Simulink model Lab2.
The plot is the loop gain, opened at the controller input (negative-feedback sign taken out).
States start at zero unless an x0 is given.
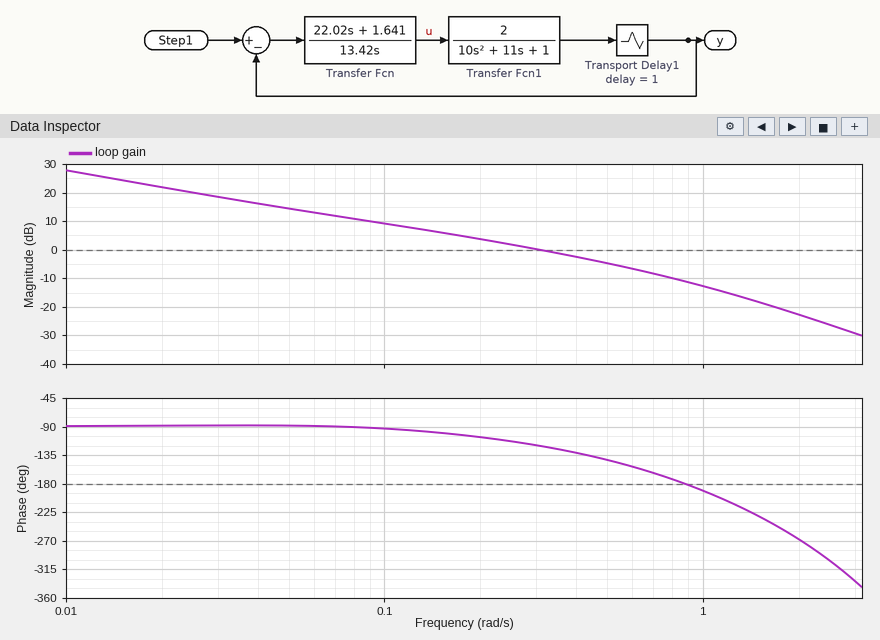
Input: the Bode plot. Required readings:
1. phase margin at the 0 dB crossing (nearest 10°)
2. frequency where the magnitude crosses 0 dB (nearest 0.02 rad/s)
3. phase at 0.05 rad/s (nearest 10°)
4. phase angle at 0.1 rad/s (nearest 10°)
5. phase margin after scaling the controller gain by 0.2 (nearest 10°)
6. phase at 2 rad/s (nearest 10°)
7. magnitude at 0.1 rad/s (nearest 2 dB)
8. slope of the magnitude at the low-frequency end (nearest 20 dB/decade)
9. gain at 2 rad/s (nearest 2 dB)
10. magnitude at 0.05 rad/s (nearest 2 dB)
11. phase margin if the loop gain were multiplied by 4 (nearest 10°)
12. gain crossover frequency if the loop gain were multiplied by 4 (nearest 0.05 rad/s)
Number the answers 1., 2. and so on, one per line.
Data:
1. 60°
2. 0.30 rad/s
3. -90°
4. -90°
5. 90°
6. -270°
7. 10 dB
8. -20 dB/decade
9. -22 dB
10. 14 dB
11. -10°
12. 0.95 rad/s
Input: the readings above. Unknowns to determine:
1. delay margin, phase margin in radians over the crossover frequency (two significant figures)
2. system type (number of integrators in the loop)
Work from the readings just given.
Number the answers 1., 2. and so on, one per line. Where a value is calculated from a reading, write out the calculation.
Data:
1. 60 × π / 180 / 0.3 = 3.5 s
2. 1
